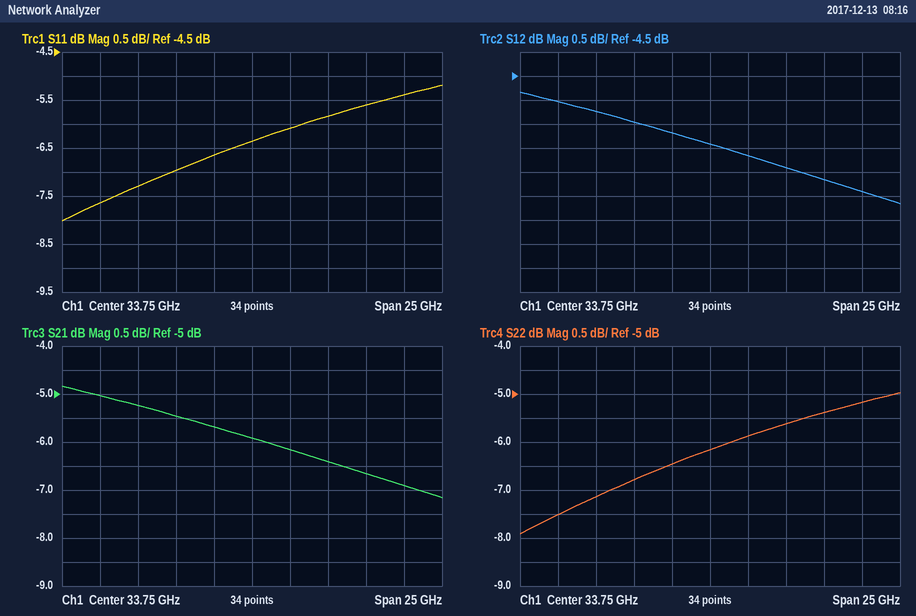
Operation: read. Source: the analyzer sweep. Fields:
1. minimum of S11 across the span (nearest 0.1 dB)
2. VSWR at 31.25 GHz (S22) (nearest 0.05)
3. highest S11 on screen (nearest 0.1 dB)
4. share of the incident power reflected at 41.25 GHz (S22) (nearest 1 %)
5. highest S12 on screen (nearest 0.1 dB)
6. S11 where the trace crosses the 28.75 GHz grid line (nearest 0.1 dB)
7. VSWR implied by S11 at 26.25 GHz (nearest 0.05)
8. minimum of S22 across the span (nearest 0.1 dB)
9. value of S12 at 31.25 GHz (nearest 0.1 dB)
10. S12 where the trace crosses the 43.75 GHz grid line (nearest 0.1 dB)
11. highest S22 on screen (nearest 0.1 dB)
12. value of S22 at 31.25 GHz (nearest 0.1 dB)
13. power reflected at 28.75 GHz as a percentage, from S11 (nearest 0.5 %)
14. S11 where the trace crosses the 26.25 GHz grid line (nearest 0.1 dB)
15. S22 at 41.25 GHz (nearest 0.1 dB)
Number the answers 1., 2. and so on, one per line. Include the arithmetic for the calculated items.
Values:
1. -8.0 dB
2. |Γ| = 10^(-6.5/20) = 0.4732; VSWR = (1 + 0.4732)/(1 − 0.4732) ≈ 2.80
3. -5.2 dB
4. 10^(-5.4/10) ≈ 29 %
5. -4.8 dB
6. -7.0 dB
7. |Γ| = 10^(-7.3/20) = 0.4315; VSWR = (1 + 0.4315)/(1 − 0.4315) ≈ 2.52, so 2.50 to the nearest 0.05
8. -7.9 dB
9. -5.7 dB
10. -6.9 dB
11. -5.0 dB
12. -6.5 dB
13. 10^(-7/10) ≈ 20.0 %
14. -7.3 dB
15. -5.4 dB
